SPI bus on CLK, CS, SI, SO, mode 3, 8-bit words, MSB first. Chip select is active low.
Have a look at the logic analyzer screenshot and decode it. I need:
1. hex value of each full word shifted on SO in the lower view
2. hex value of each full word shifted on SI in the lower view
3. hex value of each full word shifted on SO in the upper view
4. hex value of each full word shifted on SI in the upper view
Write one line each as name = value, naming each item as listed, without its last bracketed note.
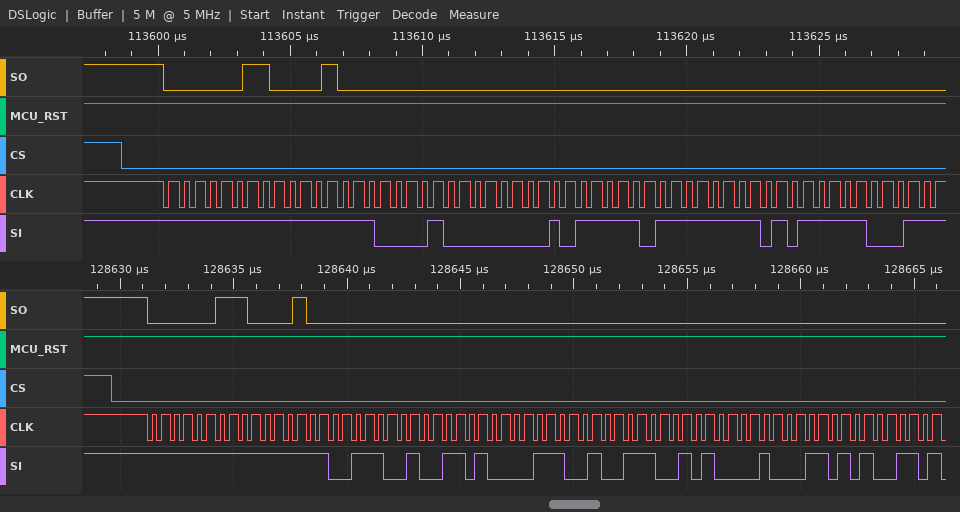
hex value of each full word shifted on SO in the lower view = 03, 84, 00, 00, 00, 00, 00, 00
hex value of each full word shifted on SI in the lower view = FF, FF, 39, 34, 39, 39, 42, 35
hex value of each full word shifted on SO in the upper view = 03, 08, 00, 00, 00, 00, 00
hex value of each full word shifted on SI in the upper view = FF, FF, 08, 05, F7, FA, F8
